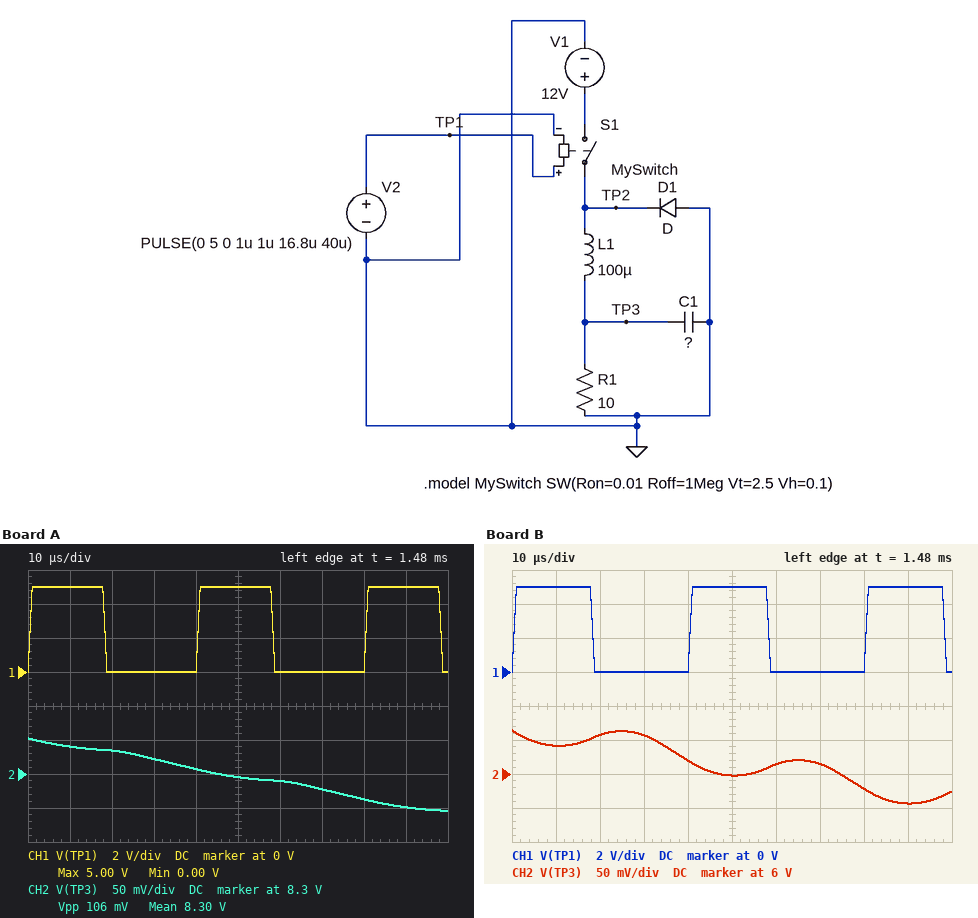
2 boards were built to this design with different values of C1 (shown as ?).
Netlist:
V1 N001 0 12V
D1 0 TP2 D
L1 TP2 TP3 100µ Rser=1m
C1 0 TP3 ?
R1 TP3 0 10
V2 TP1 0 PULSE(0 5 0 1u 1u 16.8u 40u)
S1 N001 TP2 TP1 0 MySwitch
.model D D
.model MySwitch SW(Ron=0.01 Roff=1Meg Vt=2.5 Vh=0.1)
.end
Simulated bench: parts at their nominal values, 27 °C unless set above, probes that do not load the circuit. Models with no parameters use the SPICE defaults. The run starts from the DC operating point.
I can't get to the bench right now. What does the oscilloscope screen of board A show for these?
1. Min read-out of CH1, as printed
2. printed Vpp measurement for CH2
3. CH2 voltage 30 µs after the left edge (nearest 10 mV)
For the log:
0.00 V
106 mV
8.32 V
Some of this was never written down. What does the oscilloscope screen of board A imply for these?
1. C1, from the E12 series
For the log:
560 µF
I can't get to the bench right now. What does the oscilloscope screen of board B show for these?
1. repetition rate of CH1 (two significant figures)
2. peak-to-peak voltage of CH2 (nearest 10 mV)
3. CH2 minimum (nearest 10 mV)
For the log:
25 kHz
110 mV
5.96 V
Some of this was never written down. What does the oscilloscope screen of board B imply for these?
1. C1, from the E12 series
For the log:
150 µF
